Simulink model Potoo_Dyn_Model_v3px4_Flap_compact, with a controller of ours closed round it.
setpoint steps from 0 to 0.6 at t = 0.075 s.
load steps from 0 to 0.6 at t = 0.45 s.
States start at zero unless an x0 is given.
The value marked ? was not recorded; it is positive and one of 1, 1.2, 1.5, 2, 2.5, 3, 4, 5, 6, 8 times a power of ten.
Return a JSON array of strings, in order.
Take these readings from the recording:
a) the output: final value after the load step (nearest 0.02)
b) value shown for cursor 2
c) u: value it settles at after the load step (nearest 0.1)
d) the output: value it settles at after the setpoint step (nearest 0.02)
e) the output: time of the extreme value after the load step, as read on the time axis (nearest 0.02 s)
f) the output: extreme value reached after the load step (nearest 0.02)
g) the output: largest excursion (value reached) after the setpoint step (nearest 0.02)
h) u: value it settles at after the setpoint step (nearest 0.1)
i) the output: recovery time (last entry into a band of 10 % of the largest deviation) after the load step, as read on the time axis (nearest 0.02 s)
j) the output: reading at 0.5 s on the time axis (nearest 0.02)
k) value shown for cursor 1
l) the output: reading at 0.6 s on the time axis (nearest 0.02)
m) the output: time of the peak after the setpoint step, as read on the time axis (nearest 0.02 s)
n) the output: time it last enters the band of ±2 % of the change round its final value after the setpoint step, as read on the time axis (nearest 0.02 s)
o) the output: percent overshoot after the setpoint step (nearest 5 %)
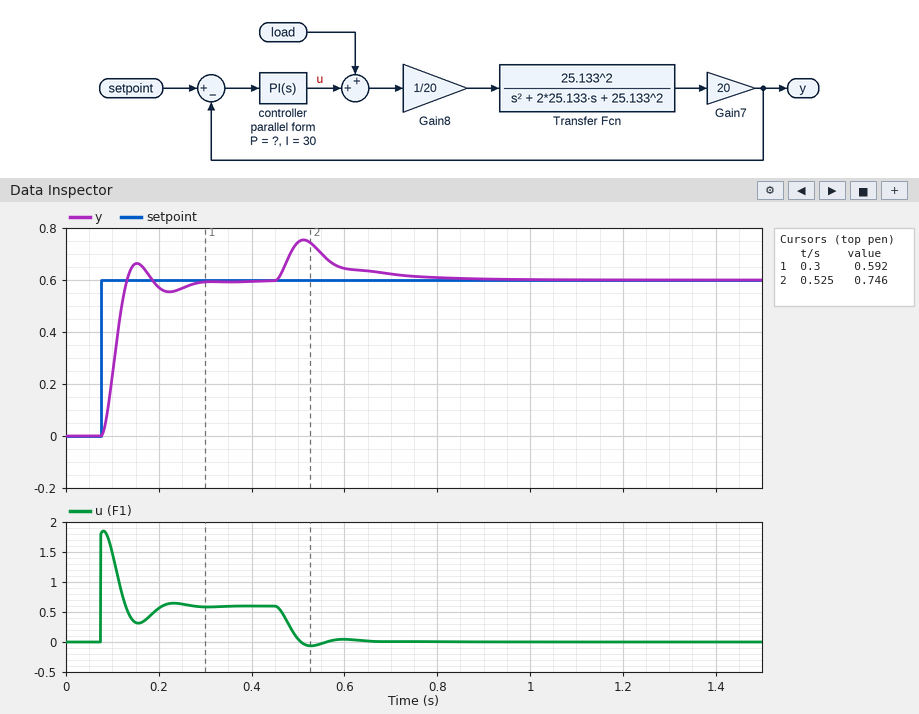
["0.60", "0.746", "0.0", "0.60", "0.52 s", "0.76", "0.66", "0.6", "0.74 s", "0.74", "0.592", "0.64", "0.16 s", "0.28 s", "10 %"]
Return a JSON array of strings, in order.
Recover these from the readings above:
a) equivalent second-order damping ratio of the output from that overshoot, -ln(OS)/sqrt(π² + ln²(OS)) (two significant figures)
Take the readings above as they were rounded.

["0.59"]
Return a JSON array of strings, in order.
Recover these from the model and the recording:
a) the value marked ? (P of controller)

["3"]
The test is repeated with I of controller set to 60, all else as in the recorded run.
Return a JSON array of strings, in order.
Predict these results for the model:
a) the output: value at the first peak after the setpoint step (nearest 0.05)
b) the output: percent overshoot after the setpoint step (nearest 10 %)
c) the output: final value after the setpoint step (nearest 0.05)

["0.80", "30 %", "0.60"]
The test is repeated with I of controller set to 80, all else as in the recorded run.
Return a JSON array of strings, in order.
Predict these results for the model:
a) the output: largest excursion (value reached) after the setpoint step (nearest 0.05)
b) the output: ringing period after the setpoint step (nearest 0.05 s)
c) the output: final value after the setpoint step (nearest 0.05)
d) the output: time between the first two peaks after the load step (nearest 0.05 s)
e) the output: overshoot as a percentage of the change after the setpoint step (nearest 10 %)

["0.85", "0.15 s", "0.60", "0.15 s", "40 %"]
